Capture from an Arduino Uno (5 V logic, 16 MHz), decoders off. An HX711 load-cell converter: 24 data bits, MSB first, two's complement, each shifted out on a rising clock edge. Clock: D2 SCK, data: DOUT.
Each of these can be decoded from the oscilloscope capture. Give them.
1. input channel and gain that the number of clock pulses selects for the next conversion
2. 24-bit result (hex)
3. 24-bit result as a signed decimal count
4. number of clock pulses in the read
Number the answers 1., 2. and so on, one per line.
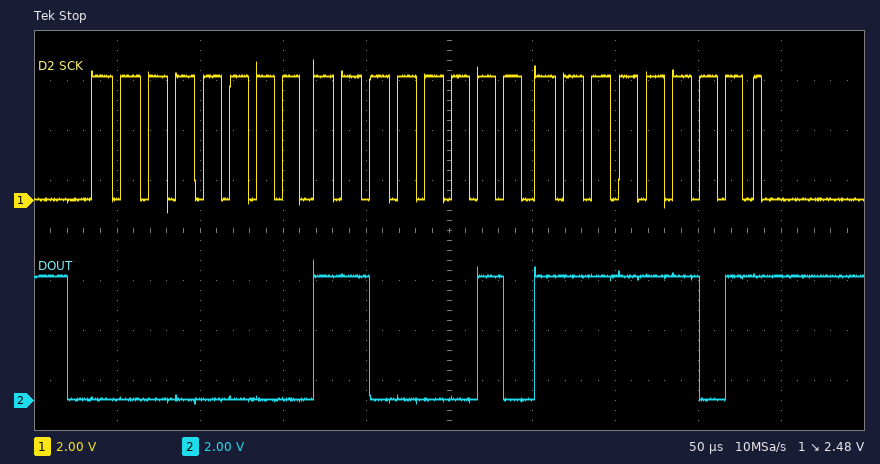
1. channel A, gain 128
2. 0x00C2FD
3. 49917
4. 25
